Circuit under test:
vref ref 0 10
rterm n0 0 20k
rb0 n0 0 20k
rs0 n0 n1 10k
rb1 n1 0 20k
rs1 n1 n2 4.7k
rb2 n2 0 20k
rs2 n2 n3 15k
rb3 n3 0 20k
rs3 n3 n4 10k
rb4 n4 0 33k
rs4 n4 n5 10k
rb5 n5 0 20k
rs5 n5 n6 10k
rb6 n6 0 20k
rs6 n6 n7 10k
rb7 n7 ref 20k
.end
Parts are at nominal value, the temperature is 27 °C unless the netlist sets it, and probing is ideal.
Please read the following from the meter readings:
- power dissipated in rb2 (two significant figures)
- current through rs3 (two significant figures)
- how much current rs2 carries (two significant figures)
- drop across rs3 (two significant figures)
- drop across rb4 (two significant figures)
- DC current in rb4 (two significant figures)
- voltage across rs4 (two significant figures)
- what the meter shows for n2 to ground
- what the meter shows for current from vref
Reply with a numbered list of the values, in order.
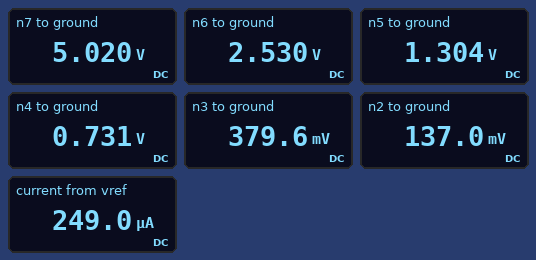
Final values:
1. 940 nW
2. 35 µA
3. 16 µA
4. 350 mV
5. 730 mV
6. 22 µA
7. 570 mV
8. 137.0 mV
9. 249.0 µA
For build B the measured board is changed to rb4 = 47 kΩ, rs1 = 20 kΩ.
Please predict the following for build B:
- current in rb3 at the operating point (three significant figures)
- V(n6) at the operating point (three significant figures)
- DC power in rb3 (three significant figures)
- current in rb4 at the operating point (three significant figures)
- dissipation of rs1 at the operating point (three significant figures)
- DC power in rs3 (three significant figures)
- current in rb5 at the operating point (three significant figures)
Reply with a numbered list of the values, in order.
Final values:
1. 21.3 µA
2. 2.55 V
3. 9.09 µW
4. 17.0 µA
5. 798 nW
6. 13.8 µW
7. 66.9 µA
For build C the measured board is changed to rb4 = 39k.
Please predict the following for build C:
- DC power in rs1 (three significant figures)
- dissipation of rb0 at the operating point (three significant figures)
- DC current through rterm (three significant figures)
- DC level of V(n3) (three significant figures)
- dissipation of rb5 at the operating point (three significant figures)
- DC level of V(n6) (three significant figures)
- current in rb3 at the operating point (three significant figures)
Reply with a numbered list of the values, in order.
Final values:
1. 440 nW
2. 117 nW
3. 2.42 µA
4. 394 mV
5. 86.9 µW
6. 2.54 V
7. 19.7 µA
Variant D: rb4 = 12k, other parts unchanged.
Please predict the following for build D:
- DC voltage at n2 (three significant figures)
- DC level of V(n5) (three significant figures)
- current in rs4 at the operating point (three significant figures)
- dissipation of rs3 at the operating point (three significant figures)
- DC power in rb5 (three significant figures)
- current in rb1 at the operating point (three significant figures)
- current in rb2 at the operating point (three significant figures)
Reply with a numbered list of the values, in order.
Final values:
1. 96.7 mV
2. 1.19 V
3. 67.8 µA
4. 6.16 µW
5. 71.3 µW
6. 3.29 µA
7. 4.84 µA
